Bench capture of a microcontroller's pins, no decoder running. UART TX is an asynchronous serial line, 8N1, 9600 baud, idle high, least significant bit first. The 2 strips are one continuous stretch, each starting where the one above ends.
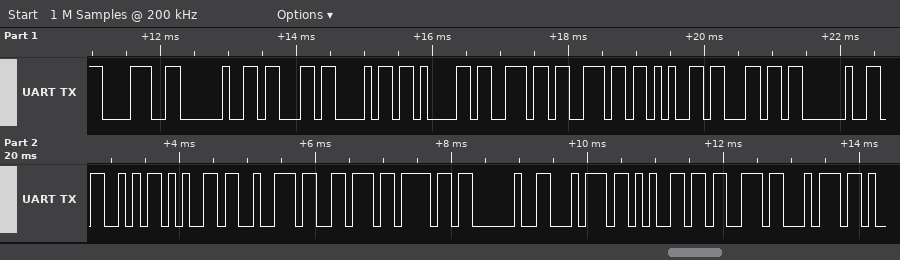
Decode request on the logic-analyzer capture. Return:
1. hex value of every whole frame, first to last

0x38 0x20 0x63 0x68 0x61 0x6E 0x6E 0x65 0x6C 0x20 0x53 0x65 0x72 0x76 0x6F 0x20 0x74 0x65 0x73 0x74
